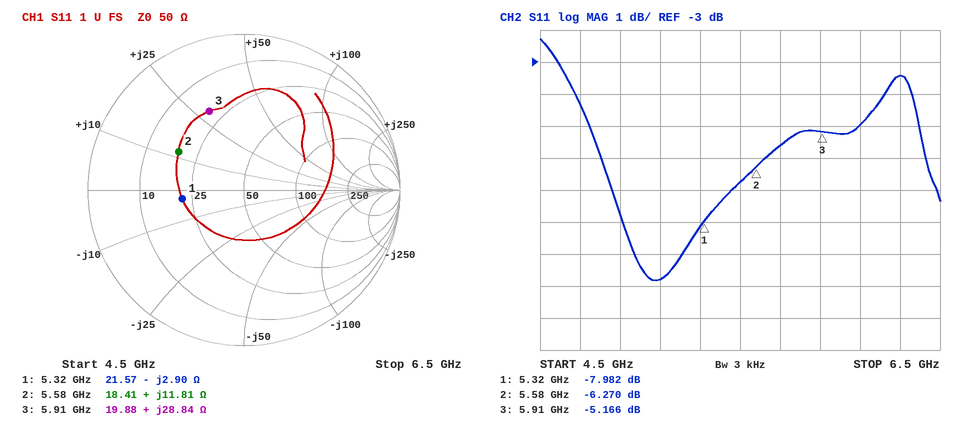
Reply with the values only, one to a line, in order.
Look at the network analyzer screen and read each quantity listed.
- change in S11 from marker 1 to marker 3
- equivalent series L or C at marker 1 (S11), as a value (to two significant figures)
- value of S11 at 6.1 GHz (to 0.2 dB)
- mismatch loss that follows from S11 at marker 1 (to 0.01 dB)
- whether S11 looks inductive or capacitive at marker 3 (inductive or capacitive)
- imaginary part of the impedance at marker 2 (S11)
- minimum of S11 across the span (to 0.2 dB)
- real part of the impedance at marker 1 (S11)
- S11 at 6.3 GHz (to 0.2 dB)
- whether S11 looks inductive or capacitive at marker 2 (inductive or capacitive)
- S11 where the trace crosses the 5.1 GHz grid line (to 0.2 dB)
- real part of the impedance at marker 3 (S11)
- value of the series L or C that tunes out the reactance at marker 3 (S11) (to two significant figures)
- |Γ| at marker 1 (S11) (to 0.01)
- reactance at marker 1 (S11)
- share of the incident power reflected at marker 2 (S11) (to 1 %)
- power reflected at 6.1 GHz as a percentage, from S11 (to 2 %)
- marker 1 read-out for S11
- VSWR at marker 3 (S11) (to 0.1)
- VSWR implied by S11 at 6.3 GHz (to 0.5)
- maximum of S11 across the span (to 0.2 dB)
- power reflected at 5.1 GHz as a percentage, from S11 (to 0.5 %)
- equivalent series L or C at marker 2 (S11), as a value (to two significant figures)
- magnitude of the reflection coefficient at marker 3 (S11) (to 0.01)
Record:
2.816 dB
10 pF
-5.0 dB
0.75 dB
inductive
+11.81 Ω
-9.8 dB
21.57 Ω
-3.4 dB
inductive
-9.8 dB
19.88 Ω
930 fF
0.40
-2.90 Ω
24 %
32 %
-7.982 dB
3.5
5.0
-2.2 dB
10.5 %
340 pH
0.55
